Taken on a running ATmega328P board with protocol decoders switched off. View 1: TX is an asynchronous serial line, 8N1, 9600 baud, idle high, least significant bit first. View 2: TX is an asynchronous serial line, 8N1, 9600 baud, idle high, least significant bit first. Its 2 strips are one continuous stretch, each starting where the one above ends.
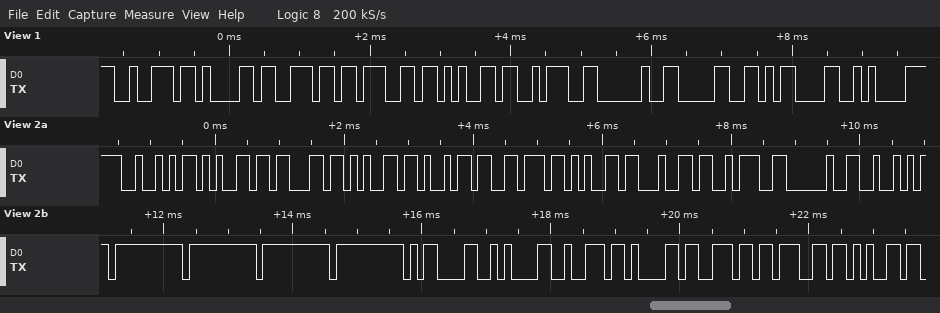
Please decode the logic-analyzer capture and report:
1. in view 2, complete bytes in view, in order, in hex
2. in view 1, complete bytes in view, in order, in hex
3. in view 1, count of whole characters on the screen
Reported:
52 65 63 65 69 76 65 64 3A 20 52 FF FF FF FF 0D 0A 72 61 6E 67 65
72 61 6E 67 65 3A 20 30 0D 0A
10
